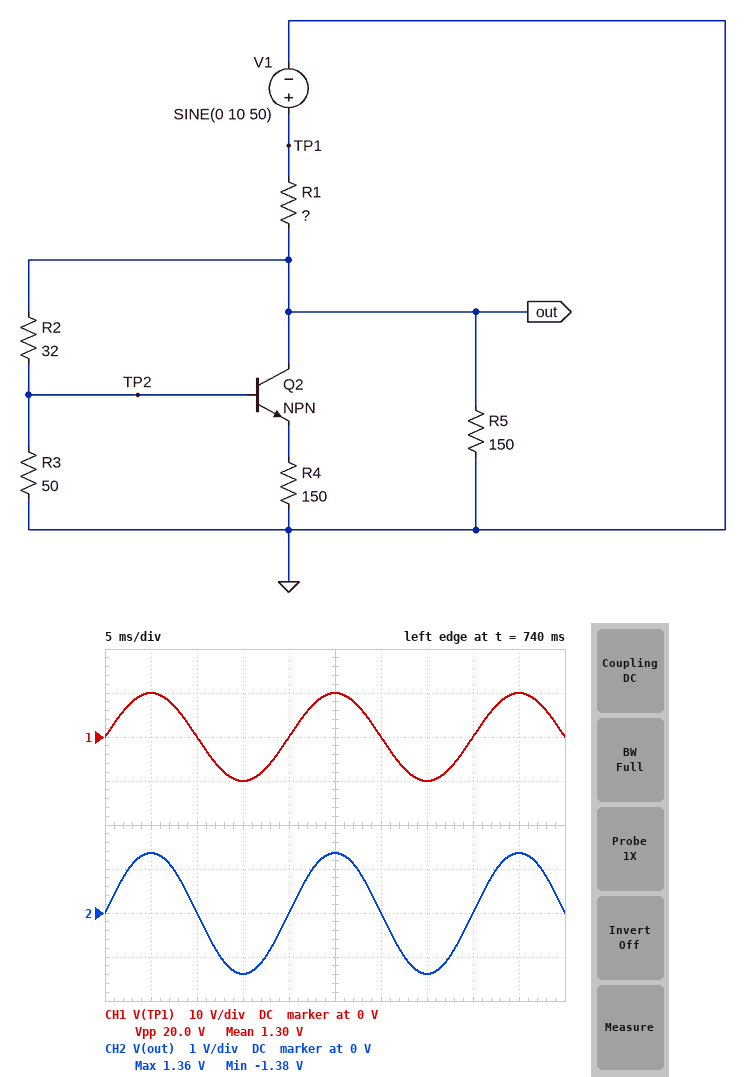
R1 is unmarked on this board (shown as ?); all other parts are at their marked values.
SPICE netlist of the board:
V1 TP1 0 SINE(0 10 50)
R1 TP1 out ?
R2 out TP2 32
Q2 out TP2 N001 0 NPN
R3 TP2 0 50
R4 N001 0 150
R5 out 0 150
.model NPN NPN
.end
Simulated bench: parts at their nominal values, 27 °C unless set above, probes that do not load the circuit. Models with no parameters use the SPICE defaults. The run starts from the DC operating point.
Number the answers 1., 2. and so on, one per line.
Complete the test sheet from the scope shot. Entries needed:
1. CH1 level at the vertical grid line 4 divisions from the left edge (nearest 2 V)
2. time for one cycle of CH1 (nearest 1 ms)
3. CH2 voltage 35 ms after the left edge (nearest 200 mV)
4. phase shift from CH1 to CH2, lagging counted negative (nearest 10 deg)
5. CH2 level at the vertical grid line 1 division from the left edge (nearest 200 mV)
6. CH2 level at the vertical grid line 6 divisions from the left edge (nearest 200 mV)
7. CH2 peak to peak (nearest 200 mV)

1. 0 V
2. 20 ms
3. -1.4 V
4. 0 deg
5. 1.4 V
6. 0 V
7. 2.8 V
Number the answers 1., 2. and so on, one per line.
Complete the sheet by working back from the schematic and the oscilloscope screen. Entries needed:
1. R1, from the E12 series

1. 330 Ω
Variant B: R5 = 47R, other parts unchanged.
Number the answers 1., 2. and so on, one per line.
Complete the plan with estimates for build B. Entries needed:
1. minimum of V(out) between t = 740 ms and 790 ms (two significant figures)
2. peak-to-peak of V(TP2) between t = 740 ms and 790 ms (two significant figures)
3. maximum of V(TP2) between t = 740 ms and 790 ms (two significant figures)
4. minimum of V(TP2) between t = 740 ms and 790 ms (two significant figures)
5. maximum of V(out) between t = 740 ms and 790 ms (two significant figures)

1. -830 mV
2. 1.0 V
3. 510 mV
4. -510 mV
5. 830 mV
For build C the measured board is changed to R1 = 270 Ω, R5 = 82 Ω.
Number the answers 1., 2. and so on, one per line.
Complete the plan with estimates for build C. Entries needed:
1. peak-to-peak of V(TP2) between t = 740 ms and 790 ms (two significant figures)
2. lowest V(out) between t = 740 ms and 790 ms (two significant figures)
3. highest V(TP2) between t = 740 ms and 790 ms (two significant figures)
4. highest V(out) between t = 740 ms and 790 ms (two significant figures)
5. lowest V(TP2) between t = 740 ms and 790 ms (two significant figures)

1. 1.6 V
2. -1.3 V
3. 800 mV
4. 1.3 V
5. -800 mV
